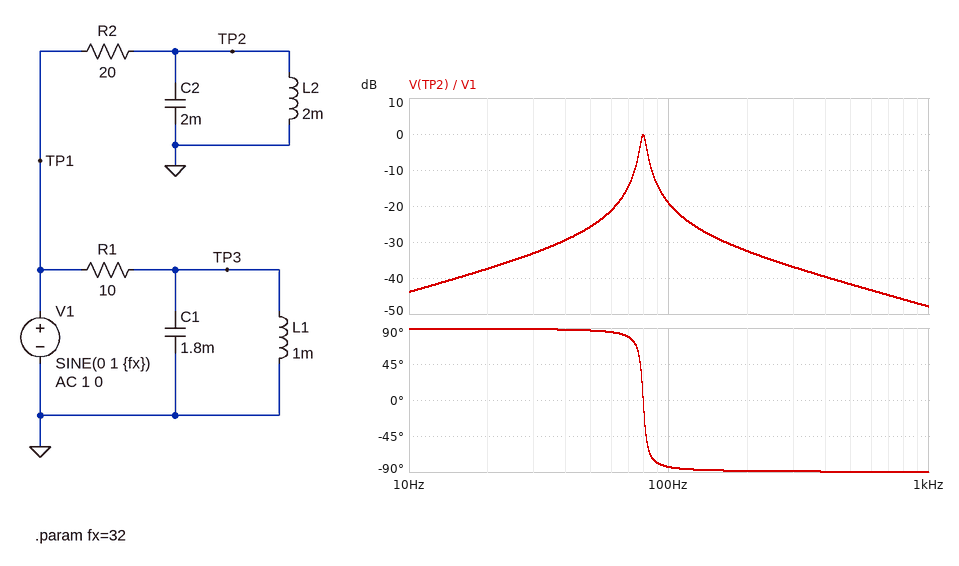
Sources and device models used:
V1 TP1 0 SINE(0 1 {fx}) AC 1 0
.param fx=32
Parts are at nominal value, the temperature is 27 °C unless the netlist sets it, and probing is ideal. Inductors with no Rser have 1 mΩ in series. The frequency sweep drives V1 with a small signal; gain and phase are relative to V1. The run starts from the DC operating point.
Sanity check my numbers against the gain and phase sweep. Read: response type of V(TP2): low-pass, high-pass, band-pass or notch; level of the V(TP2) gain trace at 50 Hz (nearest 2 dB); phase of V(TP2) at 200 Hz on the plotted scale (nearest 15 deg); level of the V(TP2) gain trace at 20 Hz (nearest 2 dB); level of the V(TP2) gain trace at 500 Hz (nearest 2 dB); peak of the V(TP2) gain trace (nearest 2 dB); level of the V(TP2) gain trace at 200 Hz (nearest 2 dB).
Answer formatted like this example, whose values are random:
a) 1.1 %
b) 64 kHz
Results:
a) band-pass
b) -26 dB
c) -90 deg
d) -38 dB
e) -42 dB
f) 0 dB
g) -32 dB
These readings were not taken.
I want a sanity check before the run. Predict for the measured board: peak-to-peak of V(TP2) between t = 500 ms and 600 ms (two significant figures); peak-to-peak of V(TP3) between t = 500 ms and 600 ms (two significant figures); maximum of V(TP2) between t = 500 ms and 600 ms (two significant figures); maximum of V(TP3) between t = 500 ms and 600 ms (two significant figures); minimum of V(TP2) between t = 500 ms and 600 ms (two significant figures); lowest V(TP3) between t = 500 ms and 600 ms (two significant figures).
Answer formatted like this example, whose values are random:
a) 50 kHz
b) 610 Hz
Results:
a) 48 mV
b) 43 mV
c) 24 mV
d) 22 mV
e) -24 mV
f) -22 mV
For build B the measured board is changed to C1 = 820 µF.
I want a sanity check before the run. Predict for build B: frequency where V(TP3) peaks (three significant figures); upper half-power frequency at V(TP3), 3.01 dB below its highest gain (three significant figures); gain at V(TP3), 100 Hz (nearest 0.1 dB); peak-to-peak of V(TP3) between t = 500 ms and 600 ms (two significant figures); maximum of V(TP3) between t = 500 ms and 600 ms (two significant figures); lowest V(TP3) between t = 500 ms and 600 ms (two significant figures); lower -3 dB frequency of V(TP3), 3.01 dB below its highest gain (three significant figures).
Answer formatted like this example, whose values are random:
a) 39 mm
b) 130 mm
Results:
a) 176 Hz
b) 186 Hz
c) -20.7 dB
d) 42 mV
e) 21 mV
f) -21 mV
g) 166 Hz
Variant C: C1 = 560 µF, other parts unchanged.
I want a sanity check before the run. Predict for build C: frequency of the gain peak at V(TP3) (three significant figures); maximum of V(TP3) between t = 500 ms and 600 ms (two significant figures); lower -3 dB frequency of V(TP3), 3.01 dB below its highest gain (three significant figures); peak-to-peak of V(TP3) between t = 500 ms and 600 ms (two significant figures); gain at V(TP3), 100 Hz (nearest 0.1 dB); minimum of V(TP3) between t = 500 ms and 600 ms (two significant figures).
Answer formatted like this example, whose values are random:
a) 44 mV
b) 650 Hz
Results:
a) 213 Hz
b) 21 mV
c) 199 Hz
d) 41 mV
e) -21.9 dB
f) -21 mV
